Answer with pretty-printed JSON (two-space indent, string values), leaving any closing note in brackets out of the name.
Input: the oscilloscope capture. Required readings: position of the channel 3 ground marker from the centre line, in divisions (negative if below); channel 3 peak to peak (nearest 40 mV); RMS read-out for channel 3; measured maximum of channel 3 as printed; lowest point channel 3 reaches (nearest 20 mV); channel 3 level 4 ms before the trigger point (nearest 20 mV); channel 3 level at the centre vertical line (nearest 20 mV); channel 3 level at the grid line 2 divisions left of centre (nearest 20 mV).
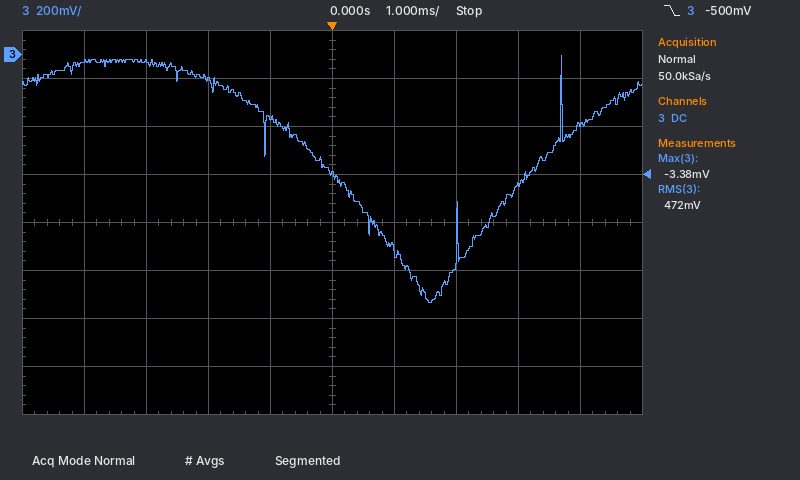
{
  "position of the channel 3 ground marker from the centre line, in divisions": "+3.5 div",
  "channel 3 peak to peak": "1.04 V",
  "RMS read-out for channel 3": "472 mV",
  "measured maximum of channel 3 as printed": "-3.38 mV",
  "lowest point channel 3 reaches": "-1.04 V",
  "channel 3 level 4 ms before the trigger point": "-20 mV",
  "channel 3 level at the centre vertical line": "-500 mV",
  "channel 3 level at the grid line 2 divisions left of centre": "-100 mV"
}
